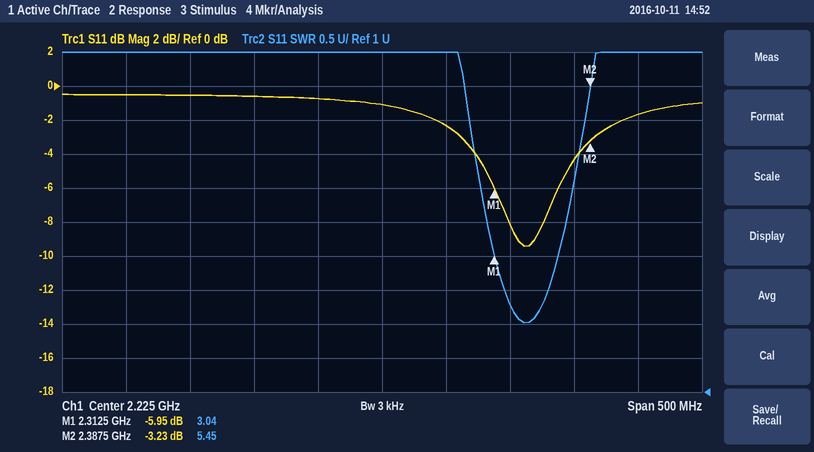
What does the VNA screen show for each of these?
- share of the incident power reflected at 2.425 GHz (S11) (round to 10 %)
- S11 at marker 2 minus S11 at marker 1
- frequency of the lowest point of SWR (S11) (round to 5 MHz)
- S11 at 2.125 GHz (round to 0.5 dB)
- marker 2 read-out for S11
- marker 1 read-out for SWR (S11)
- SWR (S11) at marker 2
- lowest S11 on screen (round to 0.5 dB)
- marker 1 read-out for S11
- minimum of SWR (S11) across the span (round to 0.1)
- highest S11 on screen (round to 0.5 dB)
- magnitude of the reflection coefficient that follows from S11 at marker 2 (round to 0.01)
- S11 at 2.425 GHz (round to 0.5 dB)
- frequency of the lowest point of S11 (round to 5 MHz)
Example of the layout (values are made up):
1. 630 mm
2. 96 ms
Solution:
1. 70 %
2. 2.72 dB
3. 2.335 GHz
4. -0.5 dB
5. -3.23 dB
6. 3.04
7. 5.45
8. -9.5 dB
9. -5.95 dB
10. 2.0
11. -0.5 dB
12. 0.69
13. -1.5 dB
14. 2.335 GHz
